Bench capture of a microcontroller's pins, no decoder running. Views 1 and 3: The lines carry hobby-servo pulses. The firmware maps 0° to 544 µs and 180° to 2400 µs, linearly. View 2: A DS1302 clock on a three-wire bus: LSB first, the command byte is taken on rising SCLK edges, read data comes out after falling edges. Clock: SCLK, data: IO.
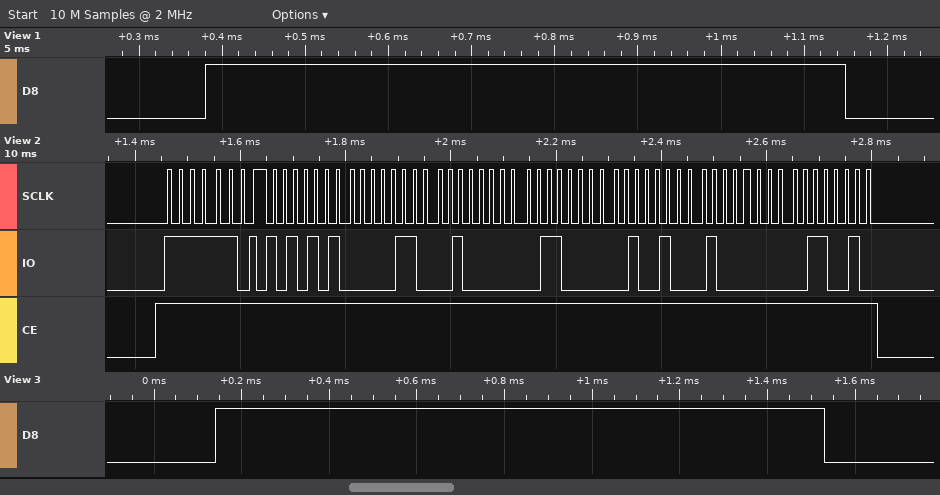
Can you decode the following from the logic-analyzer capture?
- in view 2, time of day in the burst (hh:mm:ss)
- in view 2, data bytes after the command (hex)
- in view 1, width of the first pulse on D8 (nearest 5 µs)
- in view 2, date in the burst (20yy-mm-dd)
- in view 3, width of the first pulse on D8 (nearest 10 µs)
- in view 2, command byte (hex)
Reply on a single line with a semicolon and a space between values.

02:30:55; 55 30 02 06 12 01 26; 770 µs; 2026-12-06; 1390 µs; 0xBF
